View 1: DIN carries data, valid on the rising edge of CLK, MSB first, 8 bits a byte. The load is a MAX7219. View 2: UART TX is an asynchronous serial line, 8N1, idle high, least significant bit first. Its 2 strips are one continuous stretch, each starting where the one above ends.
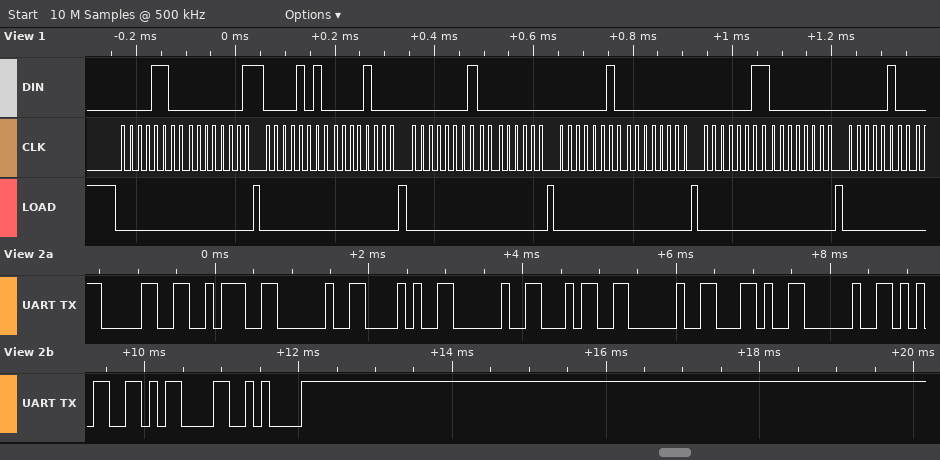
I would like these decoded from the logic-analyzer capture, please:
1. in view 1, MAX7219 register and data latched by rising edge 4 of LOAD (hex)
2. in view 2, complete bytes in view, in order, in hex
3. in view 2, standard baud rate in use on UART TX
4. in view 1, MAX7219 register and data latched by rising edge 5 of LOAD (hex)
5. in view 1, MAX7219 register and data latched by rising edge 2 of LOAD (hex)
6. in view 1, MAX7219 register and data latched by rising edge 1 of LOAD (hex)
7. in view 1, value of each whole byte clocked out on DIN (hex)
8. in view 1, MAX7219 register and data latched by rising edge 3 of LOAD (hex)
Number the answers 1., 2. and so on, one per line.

1. register 0x2, data 0x00
2. 30 3A 20 28 20 34 20 2C 20 35 0D 0A
3. 9600 baud
4. register 0x3, data 0x00
5. register 0xA, data 0x08
6. register 0xC, data 0x01
7. 0C 01 0A 08 01 00 02 00 03 00 04
8. register 0x1, data 0x00
